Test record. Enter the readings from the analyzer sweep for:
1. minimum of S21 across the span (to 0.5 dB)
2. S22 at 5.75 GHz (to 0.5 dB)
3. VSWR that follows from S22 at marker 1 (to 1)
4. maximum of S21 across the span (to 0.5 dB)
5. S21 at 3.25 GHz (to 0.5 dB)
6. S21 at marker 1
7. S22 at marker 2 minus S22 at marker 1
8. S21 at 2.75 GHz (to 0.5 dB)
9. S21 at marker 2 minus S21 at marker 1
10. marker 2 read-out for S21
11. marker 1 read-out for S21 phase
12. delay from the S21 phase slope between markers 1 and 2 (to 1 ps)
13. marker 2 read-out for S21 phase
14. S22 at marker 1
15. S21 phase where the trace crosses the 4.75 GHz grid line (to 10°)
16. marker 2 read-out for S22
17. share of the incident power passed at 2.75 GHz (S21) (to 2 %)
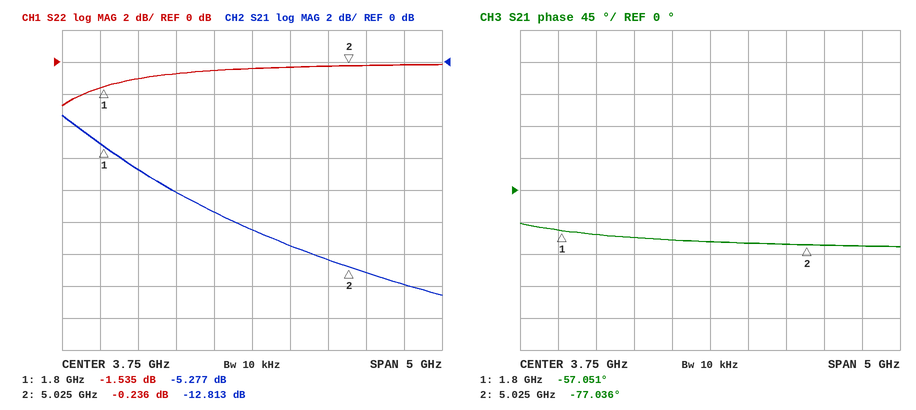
-14.5 dB
0.0 dB
11
-3.5 dB
-9.5 dB
-5.277 dB
1.299 dB
-8.0 dB
-7.536 dB
-12.813 dB
-57.051°
17 ps
-77.036°
-1.535 dB
-80°
-0.236 dB
16 %
